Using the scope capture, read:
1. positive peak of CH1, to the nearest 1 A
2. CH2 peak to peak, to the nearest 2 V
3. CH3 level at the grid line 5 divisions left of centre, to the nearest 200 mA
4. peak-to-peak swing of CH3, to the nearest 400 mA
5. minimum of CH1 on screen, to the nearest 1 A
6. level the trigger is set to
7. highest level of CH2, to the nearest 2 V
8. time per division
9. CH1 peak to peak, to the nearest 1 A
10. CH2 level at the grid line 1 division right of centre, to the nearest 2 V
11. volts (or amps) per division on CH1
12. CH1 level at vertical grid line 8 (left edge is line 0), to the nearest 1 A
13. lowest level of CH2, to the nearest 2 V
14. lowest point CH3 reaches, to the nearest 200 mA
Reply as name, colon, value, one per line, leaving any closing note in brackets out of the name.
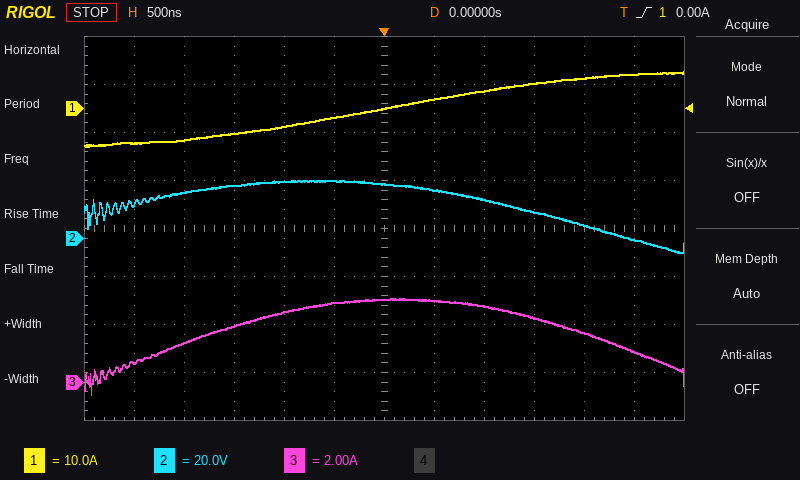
positive peak of CH1, to the nearest 1 A: 8 A
CH2 peak to peak, to the nearest 2 V: 30 V
CH3 level at the grid line 5 divisions left of centre, to the nearest 200 mA: 800 mA
peak-to-peak swing of CH3, to the nearest 400 mA: 4.0 A
minimum of CH1 on screen, to the nearest 1 A: -8 A
level the trigger is set to: 0.00 A
highest level of CH2, to the nearest 2 V: 24 V
time per division: 500 ns
CH1 peak to peak, to the nearest 1 A: 16 A
CH2 level at the grid line 1 division right of centre, to the nearest 2 V: 20 V
volts (or amps) per division on CH1: 10 A
CH1 level at vertical grid line 8 (left edge is line 0), to the nearest 1 A: 4 A
lowest level of CH2, to the nearest 2 V: -6 V
lowest point CH3 reaches, to the nearest 200 mA: -600 mA
